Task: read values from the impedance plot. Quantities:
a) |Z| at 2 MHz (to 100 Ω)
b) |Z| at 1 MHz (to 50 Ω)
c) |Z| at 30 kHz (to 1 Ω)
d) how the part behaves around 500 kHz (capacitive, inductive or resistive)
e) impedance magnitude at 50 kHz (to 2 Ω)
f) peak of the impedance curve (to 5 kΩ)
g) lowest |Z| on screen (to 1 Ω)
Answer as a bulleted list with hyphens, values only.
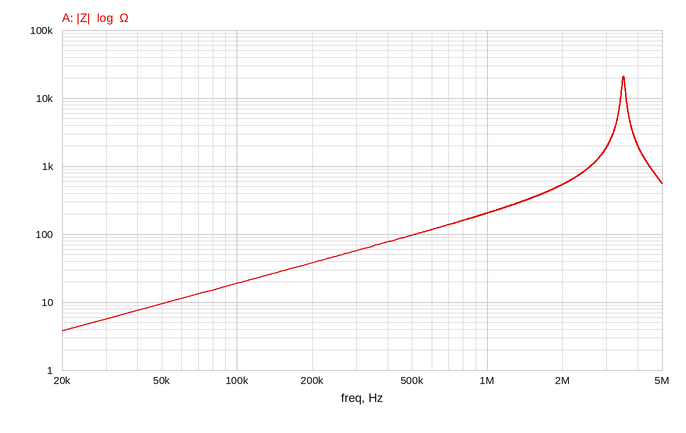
- 500 Ω
- 200 Ω
- 6 Ω
- inductive
- 10 Ω
- 20 kΩ
- 4 Ω
